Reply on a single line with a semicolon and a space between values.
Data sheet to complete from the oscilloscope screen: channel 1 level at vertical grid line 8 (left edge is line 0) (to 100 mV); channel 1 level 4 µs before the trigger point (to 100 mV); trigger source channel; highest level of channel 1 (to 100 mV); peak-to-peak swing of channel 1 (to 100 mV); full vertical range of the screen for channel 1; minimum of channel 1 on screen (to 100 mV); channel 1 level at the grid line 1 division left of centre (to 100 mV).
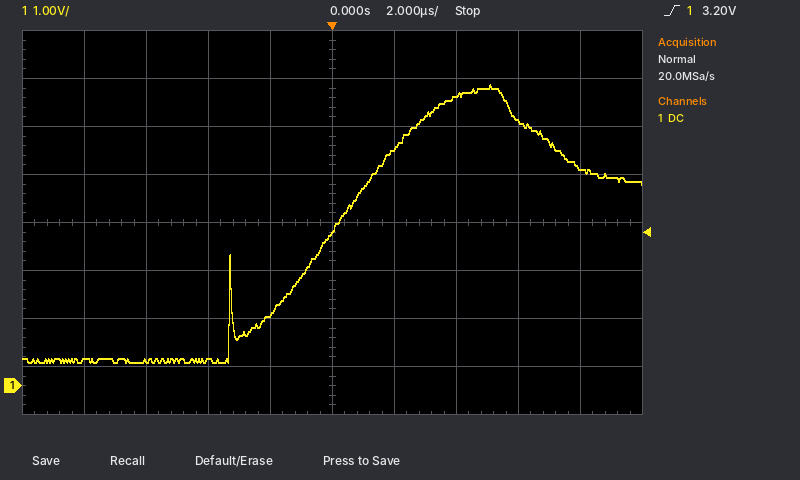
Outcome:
5.5 V; 500 mV; channel 1; 6.3 V; 5.8 V; 8 V; 500 mV; 1.5 V
